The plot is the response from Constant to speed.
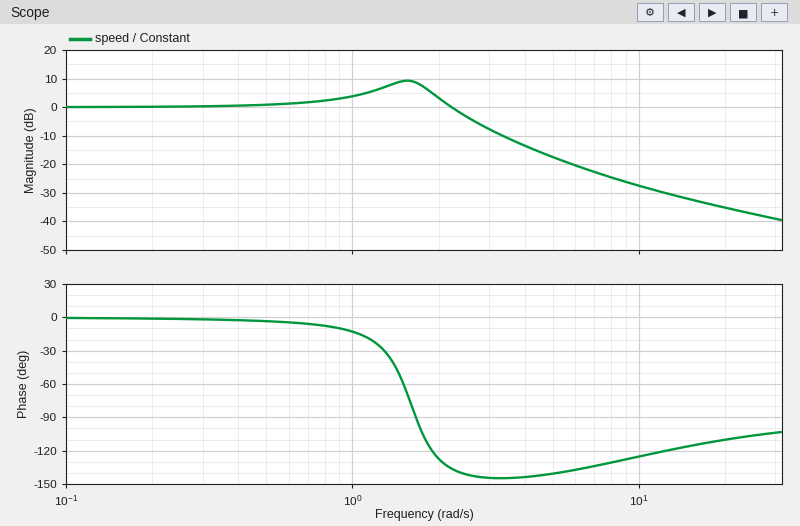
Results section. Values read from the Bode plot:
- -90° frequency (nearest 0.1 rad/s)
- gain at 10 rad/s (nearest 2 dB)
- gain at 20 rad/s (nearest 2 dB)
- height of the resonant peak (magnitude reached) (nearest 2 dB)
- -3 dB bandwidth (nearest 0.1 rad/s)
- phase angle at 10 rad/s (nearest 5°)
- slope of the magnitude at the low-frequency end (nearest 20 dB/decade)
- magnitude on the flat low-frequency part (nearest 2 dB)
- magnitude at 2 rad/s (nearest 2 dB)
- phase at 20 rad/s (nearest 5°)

1.7 rad/s
-28 dB
-36 dB
10 dB
2.5 rad/s
-125°
0 dB/decade
0 dB
4 dB
-110°
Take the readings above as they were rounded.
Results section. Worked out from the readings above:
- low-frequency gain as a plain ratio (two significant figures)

1.0
